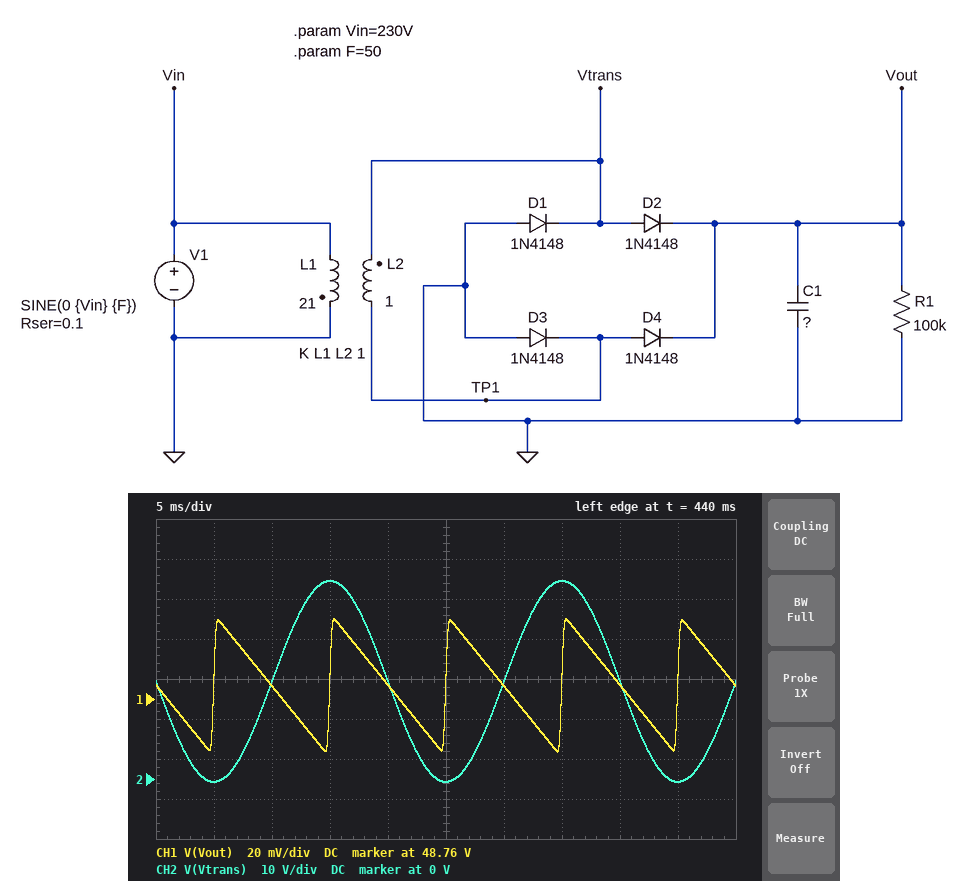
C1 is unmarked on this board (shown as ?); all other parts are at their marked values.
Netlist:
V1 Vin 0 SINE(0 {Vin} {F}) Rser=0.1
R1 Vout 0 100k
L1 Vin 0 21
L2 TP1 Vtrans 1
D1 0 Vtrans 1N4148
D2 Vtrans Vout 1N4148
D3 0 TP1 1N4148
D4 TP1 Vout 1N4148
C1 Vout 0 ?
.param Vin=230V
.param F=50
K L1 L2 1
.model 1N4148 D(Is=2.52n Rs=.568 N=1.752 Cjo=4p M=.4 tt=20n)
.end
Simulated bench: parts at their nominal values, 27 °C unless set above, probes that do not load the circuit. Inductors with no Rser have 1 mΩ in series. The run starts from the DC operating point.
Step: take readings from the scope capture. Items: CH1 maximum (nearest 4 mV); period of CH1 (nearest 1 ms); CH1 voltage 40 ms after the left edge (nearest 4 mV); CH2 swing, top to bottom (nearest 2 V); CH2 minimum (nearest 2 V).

48.800 V
10 ms
48.768 V
50 V
0 V
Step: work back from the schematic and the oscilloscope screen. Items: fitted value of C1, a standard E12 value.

68 µF
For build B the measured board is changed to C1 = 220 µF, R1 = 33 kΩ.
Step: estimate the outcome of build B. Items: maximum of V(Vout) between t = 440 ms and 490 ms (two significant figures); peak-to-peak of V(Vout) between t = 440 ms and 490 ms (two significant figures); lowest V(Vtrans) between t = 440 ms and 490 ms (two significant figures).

49 V
62 mV
-770 mV
